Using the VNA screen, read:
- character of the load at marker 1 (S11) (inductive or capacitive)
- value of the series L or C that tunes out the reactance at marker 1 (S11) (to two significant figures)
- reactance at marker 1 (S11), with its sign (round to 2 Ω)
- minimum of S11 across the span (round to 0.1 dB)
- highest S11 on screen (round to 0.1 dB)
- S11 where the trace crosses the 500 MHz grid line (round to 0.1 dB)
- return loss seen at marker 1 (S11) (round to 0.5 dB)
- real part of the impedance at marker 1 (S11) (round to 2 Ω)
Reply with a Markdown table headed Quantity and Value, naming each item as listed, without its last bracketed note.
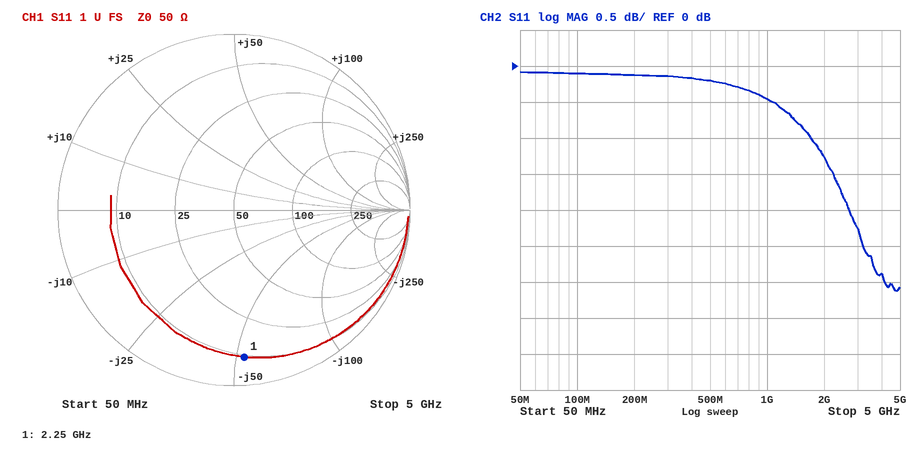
| Quantity | Value |
|---|---|
| character of the load at marker 1 (S11) | capacitive |
| value of the series L or C that tunes out the reactance at marker 1 (S11) | 3.7 nH |
| reactance at marker 1 (S11), with its sign | -52 Ω |
| minimum of S11 across the span | -3.1 dB |
| highest S11 on screen | -0.1 dB |
| S11 where the trace crosses the 500 MHz grid line | -0.2 dB |
| return loss seen at marker 1 (S11) | 1.5 dB |
| real part of the impedance at marker 1 (S11) | 10 Ω |
